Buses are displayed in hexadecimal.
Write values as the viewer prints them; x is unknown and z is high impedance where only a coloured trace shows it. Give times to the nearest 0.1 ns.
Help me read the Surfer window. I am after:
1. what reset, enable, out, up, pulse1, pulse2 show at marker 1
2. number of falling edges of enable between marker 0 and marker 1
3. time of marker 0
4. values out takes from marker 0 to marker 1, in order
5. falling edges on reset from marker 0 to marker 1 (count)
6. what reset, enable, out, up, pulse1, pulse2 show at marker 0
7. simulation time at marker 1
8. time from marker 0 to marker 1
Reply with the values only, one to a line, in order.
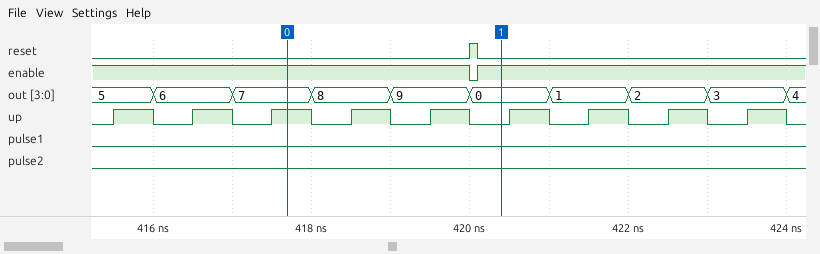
reset=0, enable=1, out=0, up=0, pulse1=0, pulse2=0
1
417.7 ns
7, 8, 9, 0
1
reset=0, enable=1, out=7, up=1, pulse1=0, pulse2=0
420.4 ns
2.7 ns
